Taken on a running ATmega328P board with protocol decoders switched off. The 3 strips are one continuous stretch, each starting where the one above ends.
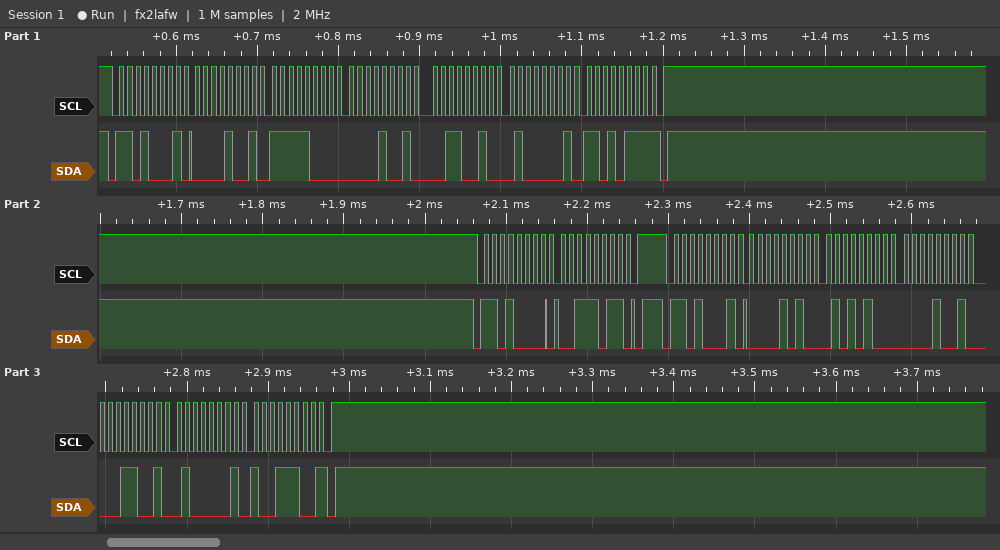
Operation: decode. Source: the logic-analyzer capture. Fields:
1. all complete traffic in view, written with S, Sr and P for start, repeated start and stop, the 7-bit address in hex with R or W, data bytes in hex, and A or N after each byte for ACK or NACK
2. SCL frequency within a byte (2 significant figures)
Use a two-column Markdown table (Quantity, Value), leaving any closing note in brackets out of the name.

| Quantity | Value |
|---|---|
| all complete traffic in view, written with S, Sr and P for start, repeated start and stop, the 7-bit address in hex with R or W, data bytes in hex, and A or N after each byte for ACK or NACK | S 68R A 09 A F8 A 09 A 32 A 41 A D7 N P S 68W A 3B A P S 68R A 0A A 54 A 09 A 19 A 41 A 9C N P |
| SCL frequency within a byte | 100 kHz |
